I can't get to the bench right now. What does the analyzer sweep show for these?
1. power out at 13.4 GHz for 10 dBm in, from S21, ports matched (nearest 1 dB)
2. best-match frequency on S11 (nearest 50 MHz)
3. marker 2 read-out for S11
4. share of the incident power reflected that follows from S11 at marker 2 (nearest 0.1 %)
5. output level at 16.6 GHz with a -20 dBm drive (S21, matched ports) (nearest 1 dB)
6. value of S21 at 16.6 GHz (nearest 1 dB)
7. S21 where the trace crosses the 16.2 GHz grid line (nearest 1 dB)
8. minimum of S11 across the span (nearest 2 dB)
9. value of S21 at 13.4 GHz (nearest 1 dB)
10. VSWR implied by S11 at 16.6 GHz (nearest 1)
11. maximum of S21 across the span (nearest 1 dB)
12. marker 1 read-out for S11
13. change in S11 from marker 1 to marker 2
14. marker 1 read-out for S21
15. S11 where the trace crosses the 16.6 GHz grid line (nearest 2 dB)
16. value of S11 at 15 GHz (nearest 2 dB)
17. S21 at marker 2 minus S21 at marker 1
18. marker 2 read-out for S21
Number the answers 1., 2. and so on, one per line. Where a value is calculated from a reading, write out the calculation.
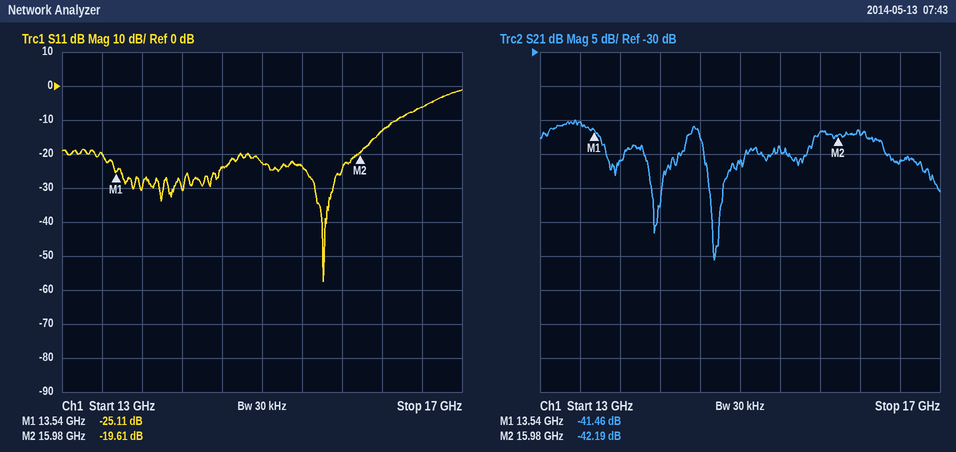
1. 10 dBm + (-40 dB) = -30 dBm
2. 15.60 GHz
3. -19.61 dB
4. 10^(-19.61/10) ≈ 1.1 %
5. -20 dBm + (-46 dB) = -66 dBm
6. -46 dB
7. -42 dB
8. -58 dB
9. -40 dB
10. |Γ| = 10^(-6/20) = 0.5012; VSWR = (1 + 0.5012)/(1 − 0.5012) ≈ 3
11. -40 dB
12. -25.11 dB
13. -19.61 − (-25.11) = 5.50 dB
14. -41.46 dB
15. -6 dB
16. -22 dB
17. -42.19 − (-41.46) = -0.73 dB
18. -42.19 dB
